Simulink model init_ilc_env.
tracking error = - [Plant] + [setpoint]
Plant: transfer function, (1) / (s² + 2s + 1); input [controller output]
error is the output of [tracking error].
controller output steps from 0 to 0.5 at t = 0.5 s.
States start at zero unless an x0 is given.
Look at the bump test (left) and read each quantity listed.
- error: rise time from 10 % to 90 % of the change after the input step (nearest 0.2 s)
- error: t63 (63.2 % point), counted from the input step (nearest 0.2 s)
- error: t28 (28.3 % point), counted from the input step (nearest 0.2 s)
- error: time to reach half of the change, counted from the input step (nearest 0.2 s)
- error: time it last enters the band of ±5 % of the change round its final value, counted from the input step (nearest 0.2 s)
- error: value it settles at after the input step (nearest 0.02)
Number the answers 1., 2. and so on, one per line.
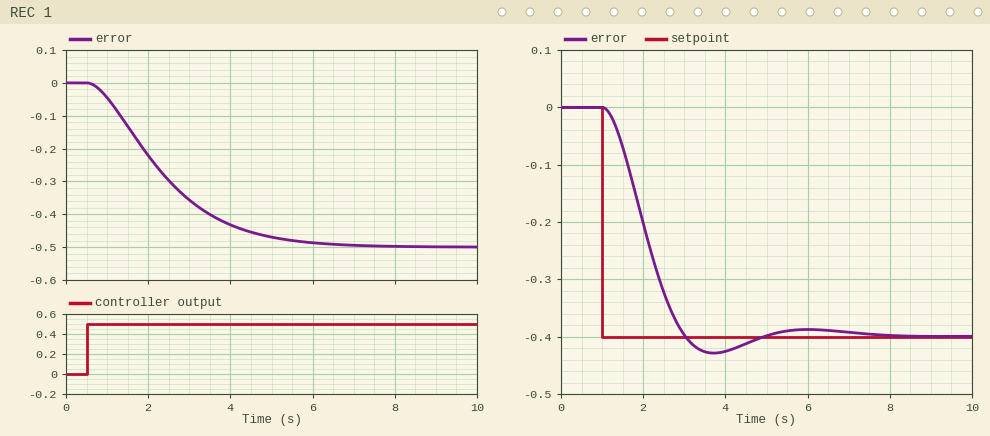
1. 3.4 s
2. 2.2 s
3. 1.0 s
4. 1.6 s
5. 4.8 s
6. -0.50
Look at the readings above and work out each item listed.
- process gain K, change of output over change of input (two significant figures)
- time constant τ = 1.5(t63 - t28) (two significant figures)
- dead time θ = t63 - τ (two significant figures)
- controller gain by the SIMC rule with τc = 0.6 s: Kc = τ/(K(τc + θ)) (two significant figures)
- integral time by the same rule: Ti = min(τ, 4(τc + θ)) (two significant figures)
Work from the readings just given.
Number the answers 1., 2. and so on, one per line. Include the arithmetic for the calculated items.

1. (-0.5 - 0) / 0.5 = -1.0
2. 1.5 × (2.2 - 1) = 1.8 s
3. 2.2 - 1.8 = 0.40 s
4. 1.8 / (-1 × (0.6 + 0.4)) = -1.8
5. min(1.8, 4 × (0.6 + 0.4)) = 1.8 s
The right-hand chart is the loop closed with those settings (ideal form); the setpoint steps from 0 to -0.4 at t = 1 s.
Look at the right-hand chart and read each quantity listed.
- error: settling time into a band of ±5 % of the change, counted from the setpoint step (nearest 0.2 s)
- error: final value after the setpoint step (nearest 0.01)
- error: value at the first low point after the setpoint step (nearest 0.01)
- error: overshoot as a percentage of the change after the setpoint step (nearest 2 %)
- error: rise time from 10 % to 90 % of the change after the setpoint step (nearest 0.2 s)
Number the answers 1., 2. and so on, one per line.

1. 3.2 s
2. -0.40
3. -0.43
4. 8 %
5. 1.4 s
